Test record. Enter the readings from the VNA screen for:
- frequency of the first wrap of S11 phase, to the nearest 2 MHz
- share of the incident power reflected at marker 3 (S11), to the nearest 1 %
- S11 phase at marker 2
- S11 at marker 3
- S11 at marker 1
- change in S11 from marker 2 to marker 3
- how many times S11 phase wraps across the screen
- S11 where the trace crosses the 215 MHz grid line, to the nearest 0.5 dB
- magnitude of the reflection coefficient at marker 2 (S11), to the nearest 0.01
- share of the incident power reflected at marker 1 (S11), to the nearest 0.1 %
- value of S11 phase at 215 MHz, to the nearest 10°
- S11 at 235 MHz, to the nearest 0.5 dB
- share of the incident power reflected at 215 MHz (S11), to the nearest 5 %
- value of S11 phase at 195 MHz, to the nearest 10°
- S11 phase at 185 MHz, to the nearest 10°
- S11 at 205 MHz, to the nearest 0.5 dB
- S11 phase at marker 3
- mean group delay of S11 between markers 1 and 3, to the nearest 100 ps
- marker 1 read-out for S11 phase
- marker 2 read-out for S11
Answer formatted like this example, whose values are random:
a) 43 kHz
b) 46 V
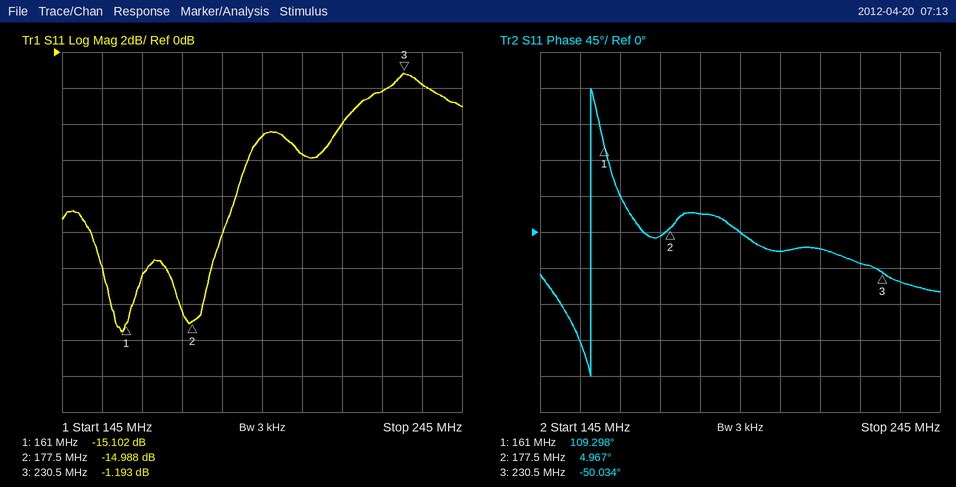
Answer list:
a) 158 MHz
b) 76 %
c) 4.967°
d) -1.193 dB
e) -15.102 dB
f) 13.795 dB
g) 1
h) -4.0 dB
i) 0.18
j) 3.1 %
k) -20°
l) -2.0 dB
m) 40 %
n) 0°
o) 20°
p) -5.5 dB
q) -50.034°
r) 6.4 ns
s) 109.298°
t) -14.988 dB
